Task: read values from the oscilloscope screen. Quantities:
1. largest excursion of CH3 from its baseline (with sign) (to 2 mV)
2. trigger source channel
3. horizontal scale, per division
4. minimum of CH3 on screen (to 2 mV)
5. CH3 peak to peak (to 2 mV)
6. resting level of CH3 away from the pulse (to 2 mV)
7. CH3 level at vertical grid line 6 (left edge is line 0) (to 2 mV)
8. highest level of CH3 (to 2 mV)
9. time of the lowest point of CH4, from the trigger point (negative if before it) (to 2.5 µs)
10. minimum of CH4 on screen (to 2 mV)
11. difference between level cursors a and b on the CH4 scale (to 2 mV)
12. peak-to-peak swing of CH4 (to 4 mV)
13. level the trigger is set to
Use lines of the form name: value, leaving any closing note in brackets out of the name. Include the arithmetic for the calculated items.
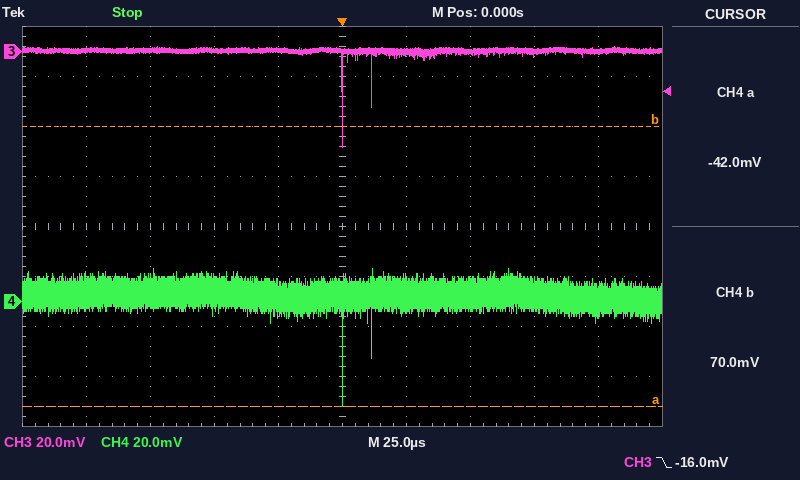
largest excursion of CH3 from its baseline (with sign): -38 mV − (0 mV) = -38 mV
trigger source channel: CH3
horizontal scale, per division: 25 µs
minimum of CH3 on screen: -38 mV
CH3 peak to peak: 2 mV − (-38 mV) = 40 mV
resting level of CH3 away from the pulse: 0 mV
CH3 level at vertical grid line 6 (left edge is line 0): 0 mV
highest level of CH3: 2 mV
time of the lowest point of CH4, from the trigger point (negative if before it): 0.0 µs
minimum of CH4 on screen: -42 mV
difference between level cursors a and b on the CH4 scale: 112 mV
peak-to-peak swing of CH4: 56 mV
level the trigger is set to: -16.0 mV
